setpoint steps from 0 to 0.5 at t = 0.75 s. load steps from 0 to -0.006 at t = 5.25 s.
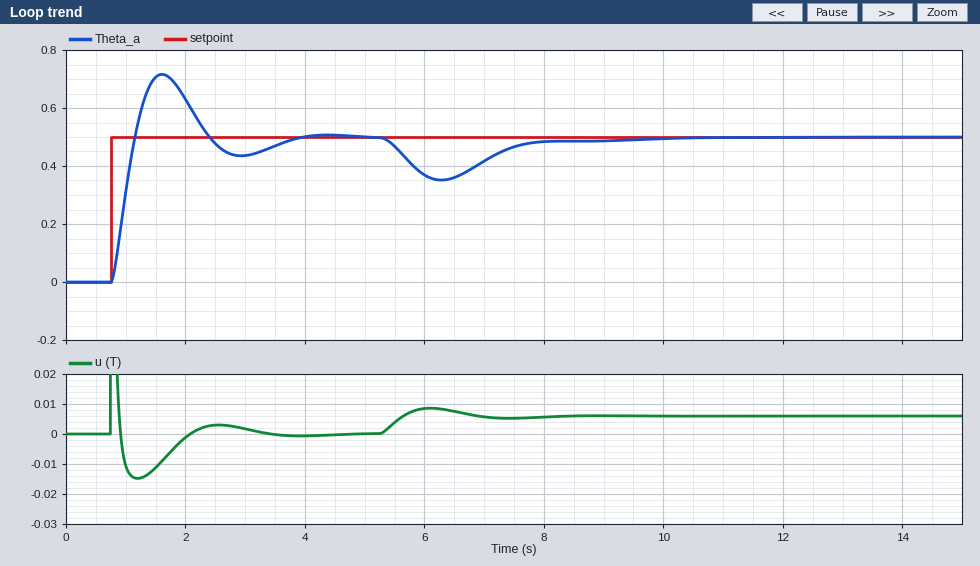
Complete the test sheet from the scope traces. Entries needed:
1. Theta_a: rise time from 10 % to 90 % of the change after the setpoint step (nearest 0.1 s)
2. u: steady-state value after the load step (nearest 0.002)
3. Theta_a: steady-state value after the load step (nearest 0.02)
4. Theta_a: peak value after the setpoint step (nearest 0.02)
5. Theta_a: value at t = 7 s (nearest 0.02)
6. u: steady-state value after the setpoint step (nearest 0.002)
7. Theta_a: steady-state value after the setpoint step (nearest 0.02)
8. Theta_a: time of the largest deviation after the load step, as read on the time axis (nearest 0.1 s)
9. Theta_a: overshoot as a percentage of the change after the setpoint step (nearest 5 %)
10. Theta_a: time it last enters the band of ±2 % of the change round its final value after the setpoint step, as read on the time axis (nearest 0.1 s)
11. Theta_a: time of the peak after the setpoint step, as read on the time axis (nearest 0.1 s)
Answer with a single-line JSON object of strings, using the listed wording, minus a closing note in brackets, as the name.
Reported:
{"Theta_a: rise time from 10 % to 90 % of the change after the setpoint step": "0.3 s", "u: steady-state value after the load step": "0.006", "Theta_a: steady-state value after the load step": "0.50", "Theta_a: peak value after the setpoint step": "0.72", "Theta_a: value at t = 7 s": "0.42", "u: steady-state value after the setpoint step": "0.000", "Theta_a: steady-state value after the setpoint step": "0.50", "Theta_a: time of the largest deviation after the load step, as read on the time axis": "6.3 s", "Theta_a: overshoot as a percentage of the change after the setpoint step": "45 %", "Theta_a: time it last enters the band of ±2 % of the change round its final value after the setpoint step, as read on the time axis": "3.8 s", "Theta_a: time of the peak after the setpoint step, as read on the time axis": "1.6 s"}
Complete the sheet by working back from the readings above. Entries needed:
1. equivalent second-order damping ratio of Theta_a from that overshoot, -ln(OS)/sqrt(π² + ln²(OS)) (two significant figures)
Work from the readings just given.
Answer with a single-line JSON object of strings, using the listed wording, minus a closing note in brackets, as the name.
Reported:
{"equivalent second-order damping ratio of Theta_a from that overshoot, -ln(OS)/sqrt(π² + ln²(OS))": "0.25"}
